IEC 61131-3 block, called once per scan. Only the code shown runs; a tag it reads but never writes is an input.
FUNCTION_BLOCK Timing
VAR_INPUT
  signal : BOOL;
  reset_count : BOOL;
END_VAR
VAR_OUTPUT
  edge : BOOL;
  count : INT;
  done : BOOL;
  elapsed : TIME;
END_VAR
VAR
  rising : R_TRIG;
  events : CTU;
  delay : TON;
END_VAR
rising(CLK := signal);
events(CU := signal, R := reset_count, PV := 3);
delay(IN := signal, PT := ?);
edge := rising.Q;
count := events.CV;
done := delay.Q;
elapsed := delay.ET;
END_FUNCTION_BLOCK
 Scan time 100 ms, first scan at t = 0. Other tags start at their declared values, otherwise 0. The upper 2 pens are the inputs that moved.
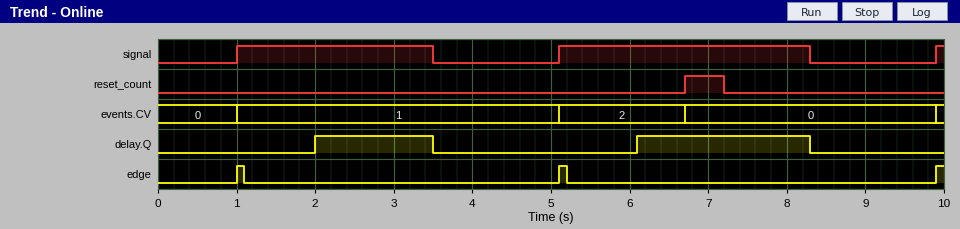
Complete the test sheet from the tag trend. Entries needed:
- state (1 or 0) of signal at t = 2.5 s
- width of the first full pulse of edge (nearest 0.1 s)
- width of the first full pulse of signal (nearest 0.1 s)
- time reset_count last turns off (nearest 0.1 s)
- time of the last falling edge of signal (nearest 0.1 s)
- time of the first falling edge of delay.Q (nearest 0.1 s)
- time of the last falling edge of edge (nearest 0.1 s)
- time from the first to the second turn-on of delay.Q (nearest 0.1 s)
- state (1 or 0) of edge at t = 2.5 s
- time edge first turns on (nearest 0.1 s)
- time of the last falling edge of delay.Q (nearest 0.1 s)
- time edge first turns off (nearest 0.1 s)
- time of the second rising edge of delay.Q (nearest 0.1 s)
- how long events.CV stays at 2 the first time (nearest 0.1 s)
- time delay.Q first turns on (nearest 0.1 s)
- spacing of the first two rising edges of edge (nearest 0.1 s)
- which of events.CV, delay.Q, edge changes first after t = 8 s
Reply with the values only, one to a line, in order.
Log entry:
1
0.1 s
2.5 s
7.2 s
8.3 s
3.5 s
5.2 s
4.1 s
0
1.0 s
8.3 s
1.1 s
6.1 s
1.6 s
2.0 s
4.1 s
delay.Q
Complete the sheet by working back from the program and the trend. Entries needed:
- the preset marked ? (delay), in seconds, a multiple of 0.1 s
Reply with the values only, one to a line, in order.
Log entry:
1.0 s
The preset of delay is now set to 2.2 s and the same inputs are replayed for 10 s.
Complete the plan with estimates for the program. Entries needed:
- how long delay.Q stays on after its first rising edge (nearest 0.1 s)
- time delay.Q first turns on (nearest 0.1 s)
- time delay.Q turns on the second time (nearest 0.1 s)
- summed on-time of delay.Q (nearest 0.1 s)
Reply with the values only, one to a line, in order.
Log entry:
0.3 s
3.2 s
7.3 s
1.3 s
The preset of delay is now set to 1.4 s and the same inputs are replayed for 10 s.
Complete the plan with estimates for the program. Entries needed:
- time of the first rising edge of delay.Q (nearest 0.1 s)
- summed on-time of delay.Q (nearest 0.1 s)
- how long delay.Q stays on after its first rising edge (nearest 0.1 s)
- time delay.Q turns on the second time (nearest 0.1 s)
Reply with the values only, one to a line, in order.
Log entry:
2.4 s
2.9 s
1.1 s
6.5 s
